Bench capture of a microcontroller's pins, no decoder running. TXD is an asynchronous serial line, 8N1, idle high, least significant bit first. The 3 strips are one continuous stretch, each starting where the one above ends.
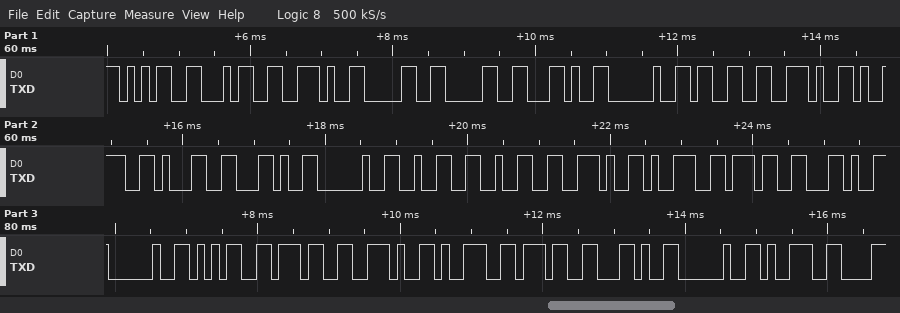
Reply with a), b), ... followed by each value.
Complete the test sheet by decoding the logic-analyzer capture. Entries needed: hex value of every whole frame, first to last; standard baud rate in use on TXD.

a) 35 34 2E 30 30 2C 20 33 2E 39 31 2C 20 32 32 2E 39 37 2C 20 35 37 2E 39 37 2C 20 39
b) 9600 baud
